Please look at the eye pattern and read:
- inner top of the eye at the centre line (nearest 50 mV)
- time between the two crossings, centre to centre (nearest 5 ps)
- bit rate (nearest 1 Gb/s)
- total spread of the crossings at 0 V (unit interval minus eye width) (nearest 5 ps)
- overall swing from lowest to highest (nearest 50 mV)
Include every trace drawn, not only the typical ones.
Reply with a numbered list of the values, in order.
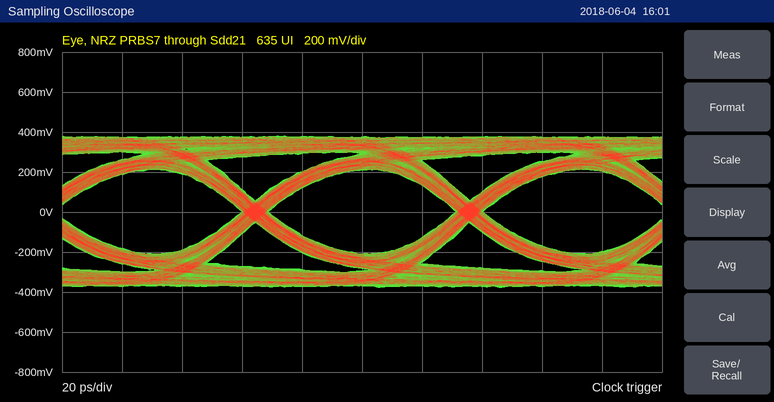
1. 200 mV
2. 70 ps
3. 14 Gb/s
4. 10 ps
5. 750 mV
